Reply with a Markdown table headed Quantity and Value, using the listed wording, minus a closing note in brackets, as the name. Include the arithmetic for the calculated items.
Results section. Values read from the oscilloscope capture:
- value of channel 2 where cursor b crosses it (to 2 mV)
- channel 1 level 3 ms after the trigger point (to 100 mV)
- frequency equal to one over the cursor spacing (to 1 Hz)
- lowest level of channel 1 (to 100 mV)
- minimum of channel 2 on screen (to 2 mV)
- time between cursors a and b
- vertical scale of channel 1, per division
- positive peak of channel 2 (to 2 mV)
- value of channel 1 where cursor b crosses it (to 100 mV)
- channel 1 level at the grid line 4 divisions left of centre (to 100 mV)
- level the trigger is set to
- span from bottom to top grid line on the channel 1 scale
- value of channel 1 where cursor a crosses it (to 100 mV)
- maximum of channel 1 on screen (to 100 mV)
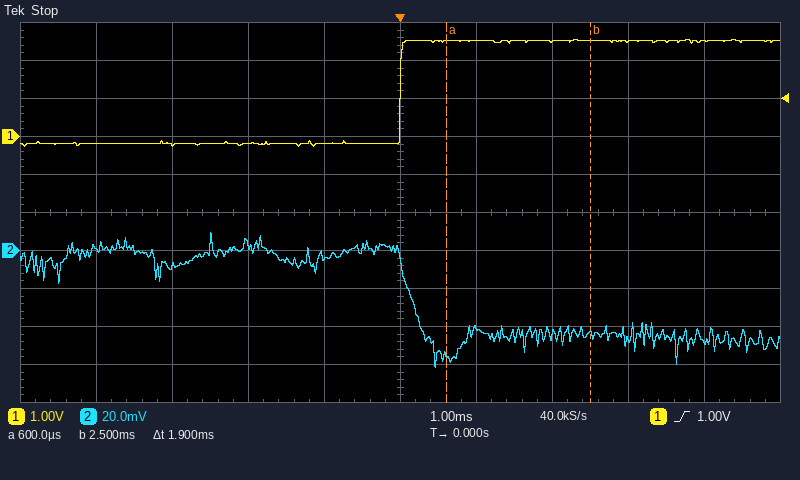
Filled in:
| Quantity | Value |
|---|---|
| value of channel 2 where cursor b crosses it | -44 mV |
| channel 1 level 3 ms after the trigger point | 2.5 V |
| frequency equal to one over the cursor spacing | 1 / 1.9 ms ≈ 526 Hz |
| lowest level of channel 1 | -300 mV |
| minimum of channel 2 on screen | -62 mV |
| time between cursors a and b | 1.9 ms |
| vertical scale of channel 1, per division | 1 V |
| positive peak of channel 2 | 10 mV |
| value of channel 1 where cursor b crosses it | 2.5 V |
| channel 1 level at the grid line 4 divisions left of centre | -200 mV |
| level the trigger is set to | 1.00 V |
| span from bottom to top grid line on the channel 1 scale | 10 V |
| value of channel 1 where cursor a crosses it | 2.5 V |
| maximum of channel 1 on screen | 2.6 V |
